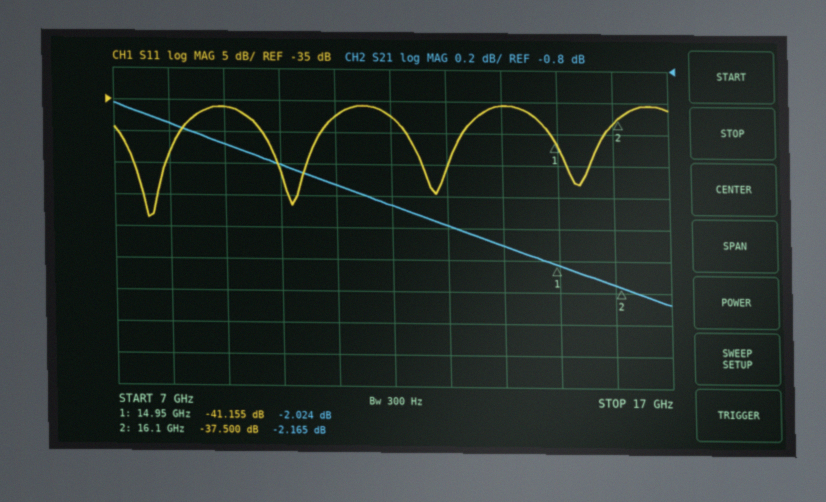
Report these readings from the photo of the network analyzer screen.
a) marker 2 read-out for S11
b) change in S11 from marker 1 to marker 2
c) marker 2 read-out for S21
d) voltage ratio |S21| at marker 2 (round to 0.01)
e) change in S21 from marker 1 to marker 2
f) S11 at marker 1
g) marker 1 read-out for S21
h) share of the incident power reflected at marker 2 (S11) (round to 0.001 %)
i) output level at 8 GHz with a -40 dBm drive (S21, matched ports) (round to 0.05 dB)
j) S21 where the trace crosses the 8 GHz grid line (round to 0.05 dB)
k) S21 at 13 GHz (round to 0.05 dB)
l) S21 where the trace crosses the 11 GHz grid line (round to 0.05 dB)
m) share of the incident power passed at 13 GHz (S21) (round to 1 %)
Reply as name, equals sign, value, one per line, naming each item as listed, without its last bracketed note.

marker 2 read-out for S11 = -37.500 dB
change in S11 from marker 1 to marker 2 = 3.655 dB
marker 2 read-out for S21 = -2.165 dB
voltage ratio |S21| at marker 2 = 0.78
change in S21 from marker 1 to marker 2 = -0.141 dB
S11 at marker 1 = -41.155 dB
marker 1 read-out for S21 = -2.024 dB
share of the incident power reflected at marker 2 (S11) = 0.018 %
output level at 8 GHz with a -40 dBm drive (S21, matched ports) = -41.15 dBm
S21 where the trace crosses the 8 GHz grid line = -1.15 dB
S21 at 13 GHz = -1.80 dB
S21 where the trace crosses the 11 GHz grid line = -1.55 dB
share of the incident power passed at 13 GHz (S21) = 66 %
